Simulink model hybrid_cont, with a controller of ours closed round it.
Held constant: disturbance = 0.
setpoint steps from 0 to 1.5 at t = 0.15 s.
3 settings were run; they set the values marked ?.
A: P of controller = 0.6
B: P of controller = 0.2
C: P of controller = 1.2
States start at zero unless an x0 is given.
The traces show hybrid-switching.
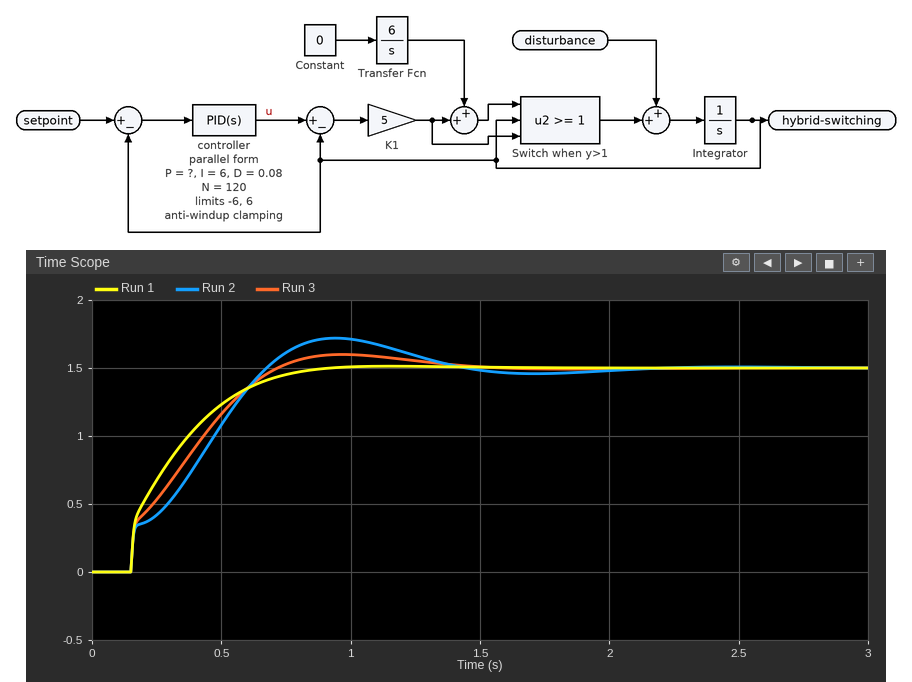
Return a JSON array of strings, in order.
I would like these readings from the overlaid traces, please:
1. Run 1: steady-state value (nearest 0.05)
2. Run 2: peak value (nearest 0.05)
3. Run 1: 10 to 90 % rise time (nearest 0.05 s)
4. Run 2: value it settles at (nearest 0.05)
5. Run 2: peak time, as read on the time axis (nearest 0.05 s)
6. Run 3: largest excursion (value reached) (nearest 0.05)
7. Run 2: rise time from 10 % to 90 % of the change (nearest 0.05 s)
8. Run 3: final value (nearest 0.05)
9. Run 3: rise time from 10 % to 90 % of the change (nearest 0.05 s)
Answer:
["1.50", "1.70", "0.45 s", "1.50", "0.95 s", "1.60", "0.45 s", "1.50", "0.45 s"]
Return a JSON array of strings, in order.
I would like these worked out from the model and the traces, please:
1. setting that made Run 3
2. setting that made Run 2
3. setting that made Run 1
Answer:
["A", "B", "C"]
